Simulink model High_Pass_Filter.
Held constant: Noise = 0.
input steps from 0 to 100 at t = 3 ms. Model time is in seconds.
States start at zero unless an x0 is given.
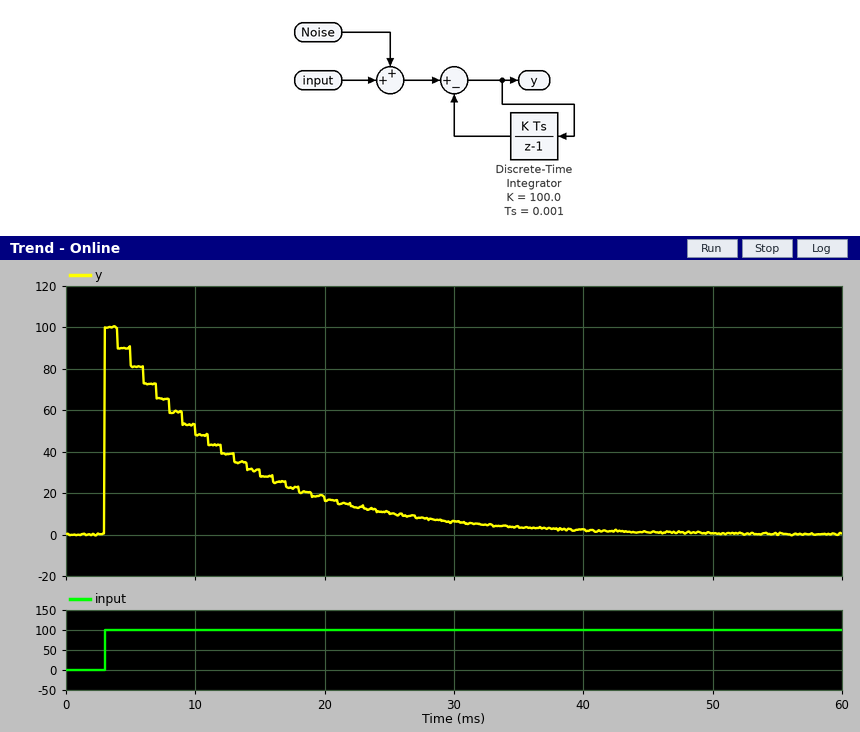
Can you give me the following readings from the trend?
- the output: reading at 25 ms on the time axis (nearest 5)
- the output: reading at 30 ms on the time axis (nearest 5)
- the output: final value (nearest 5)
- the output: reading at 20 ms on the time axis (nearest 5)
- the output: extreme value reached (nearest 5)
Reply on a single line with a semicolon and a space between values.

10; 5; 0; 15; 100
